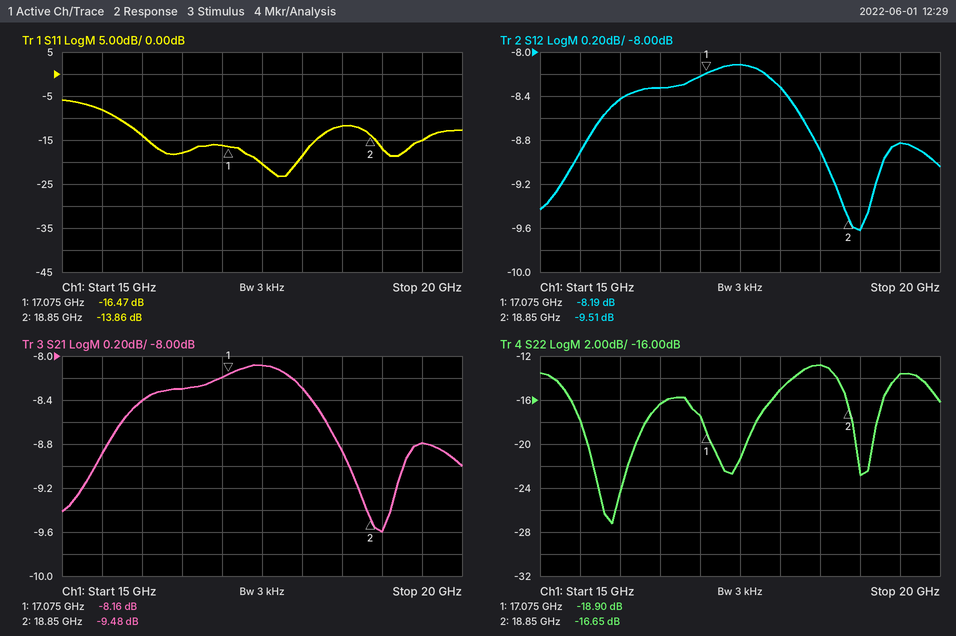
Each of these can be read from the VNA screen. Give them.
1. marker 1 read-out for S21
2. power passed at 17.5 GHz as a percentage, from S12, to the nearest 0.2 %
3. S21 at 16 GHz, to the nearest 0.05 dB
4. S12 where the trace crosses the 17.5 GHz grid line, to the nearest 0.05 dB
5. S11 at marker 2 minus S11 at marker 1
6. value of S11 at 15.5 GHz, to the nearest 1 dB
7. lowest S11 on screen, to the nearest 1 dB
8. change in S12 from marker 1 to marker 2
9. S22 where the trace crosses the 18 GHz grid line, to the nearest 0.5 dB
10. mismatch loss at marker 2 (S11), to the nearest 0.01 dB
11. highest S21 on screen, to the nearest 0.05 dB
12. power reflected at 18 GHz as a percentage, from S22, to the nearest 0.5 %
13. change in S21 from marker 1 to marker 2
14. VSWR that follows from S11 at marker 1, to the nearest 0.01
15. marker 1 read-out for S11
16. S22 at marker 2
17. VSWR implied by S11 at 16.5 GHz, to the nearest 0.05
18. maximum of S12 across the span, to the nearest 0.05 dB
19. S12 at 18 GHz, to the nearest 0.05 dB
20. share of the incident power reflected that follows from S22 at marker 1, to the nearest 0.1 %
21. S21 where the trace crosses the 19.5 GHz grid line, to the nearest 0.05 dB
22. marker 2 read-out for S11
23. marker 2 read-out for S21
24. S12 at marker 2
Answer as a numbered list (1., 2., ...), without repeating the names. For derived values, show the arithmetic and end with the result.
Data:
1. -8.16 dB
2. 10^(-8.1/10) ≈ 15.5 %, so 15.4 % to the nearest 0.2 %
3. -8.40 dB
4. -8.10 dB
5. -13.86 − (-16.47) = 2.61 dB
6. -8 dB
7. -23 dB
8. -9.51 − (-8.19) = -1.32 dB
9. -15.0 dB
10. −10 log10(1 − 10^(-13.86/10)) ≈ 0.18 dB
11. -8.10 dB
12. 10^(-15/10) ≈ 3.16 %, so 3.0 % to the nearest 0.5 %
13. -9.48 − (-8.16) = -1.32 dB
14. (1 + 0.1501)/(1 − 0.1501) ≈ 1.35
15. -16.47 dB
16. -16.65 dB
17. |Γ| = 10^(-18/20) = 0.1259; VSWR = (1 + 0.1259)/(1 − 0.1259) ≈ 1.29, so 1.30 to the nearest 0.05
18. -8.10 dB
19. -8.30 dB
20. 10^(-18.9/10) ≈ 1.3 %
21. -8.80 dB
22. -13.86 dB
23. -9.48 dB
24. -9.51 dB
